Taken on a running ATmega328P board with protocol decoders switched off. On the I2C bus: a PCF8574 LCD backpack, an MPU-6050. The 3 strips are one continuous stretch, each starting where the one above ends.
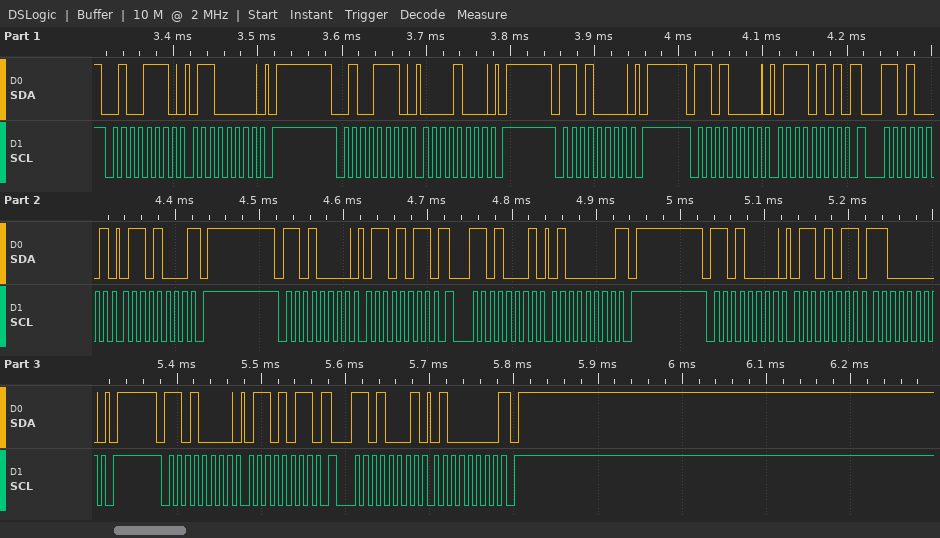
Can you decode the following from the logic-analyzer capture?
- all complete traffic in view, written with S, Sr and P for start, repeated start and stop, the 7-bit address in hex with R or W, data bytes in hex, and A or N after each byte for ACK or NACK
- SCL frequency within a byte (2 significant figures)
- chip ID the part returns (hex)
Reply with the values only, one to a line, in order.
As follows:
S 27W A 60 A P S 27W A 08 A P S 68W A P S 68W A 75 A Sr 68R A 68 N P S 68W A 6B A Sr 68R A 40 N P S 68W A 6B A C0 A P S 68W A 6B A Sr 68R A 40 N P
100 kHz
0x68
